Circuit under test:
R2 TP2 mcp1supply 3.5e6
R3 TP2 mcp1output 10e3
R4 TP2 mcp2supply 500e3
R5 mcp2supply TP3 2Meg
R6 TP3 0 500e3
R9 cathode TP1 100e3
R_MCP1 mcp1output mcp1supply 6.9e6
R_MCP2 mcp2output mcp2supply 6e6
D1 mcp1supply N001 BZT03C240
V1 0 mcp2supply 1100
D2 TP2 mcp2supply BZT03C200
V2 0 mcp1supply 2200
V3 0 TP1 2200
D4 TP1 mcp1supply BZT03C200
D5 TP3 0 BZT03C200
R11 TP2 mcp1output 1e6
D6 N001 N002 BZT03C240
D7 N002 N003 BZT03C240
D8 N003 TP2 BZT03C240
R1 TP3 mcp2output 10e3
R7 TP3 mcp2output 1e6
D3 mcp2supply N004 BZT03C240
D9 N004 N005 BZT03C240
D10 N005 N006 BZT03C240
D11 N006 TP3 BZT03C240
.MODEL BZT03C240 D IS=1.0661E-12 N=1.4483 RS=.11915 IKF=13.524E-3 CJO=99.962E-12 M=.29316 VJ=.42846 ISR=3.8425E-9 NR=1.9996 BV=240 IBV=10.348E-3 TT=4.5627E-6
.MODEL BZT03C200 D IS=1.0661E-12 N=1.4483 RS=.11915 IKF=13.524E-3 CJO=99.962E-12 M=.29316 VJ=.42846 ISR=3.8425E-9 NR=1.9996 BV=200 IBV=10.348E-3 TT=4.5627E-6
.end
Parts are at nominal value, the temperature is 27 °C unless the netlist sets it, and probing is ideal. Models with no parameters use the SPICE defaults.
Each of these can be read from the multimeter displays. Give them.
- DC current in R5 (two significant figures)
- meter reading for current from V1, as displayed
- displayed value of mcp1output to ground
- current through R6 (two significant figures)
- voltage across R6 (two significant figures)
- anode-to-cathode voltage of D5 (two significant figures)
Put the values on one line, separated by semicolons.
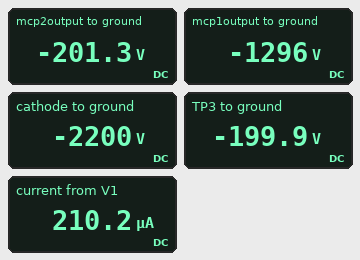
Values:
450 µA; 210.2 µA; -1296 V; 400 µA; 200 V; -200 V
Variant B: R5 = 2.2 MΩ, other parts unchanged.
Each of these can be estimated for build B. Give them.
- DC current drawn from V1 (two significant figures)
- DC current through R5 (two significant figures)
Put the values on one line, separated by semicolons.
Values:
170 µA; 410 µA
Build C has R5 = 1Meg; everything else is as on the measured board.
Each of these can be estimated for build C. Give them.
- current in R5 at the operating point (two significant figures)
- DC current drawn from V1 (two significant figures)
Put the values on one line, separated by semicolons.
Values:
900 µA; 660 µA
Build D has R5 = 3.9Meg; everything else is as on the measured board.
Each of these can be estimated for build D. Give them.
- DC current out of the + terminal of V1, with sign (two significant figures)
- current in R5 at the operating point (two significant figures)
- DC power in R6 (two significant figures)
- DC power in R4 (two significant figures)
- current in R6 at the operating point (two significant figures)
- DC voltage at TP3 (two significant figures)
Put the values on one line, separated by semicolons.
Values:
-5.7 µA; 230 µA; 74 mW; 76 mW; 380 µA; -190 V
